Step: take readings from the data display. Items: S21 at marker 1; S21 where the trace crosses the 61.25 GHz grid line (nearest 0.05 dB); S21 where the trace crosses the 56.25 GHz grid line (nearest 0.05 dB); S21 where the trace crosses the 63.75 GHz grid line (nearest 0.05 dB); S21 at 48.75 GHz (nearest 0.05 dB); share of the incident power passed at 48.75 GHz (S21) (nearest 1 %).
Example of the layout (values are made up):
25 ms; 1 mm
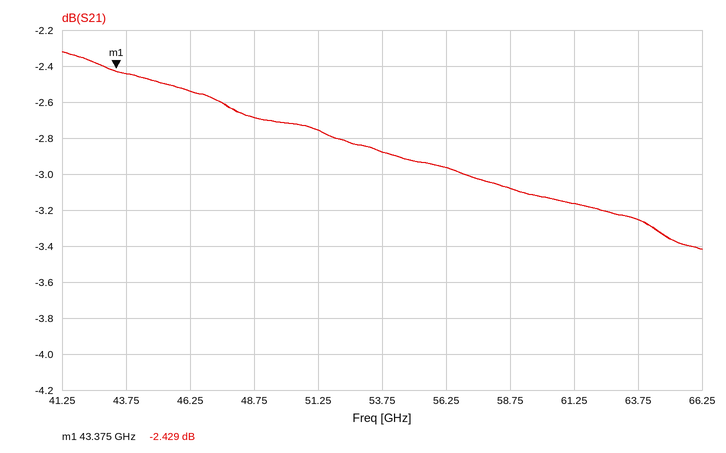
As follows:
-2.429 dB; -3.15 dB; -2.95 dB; -3.25 dB; -2.70 dB; 54 %
